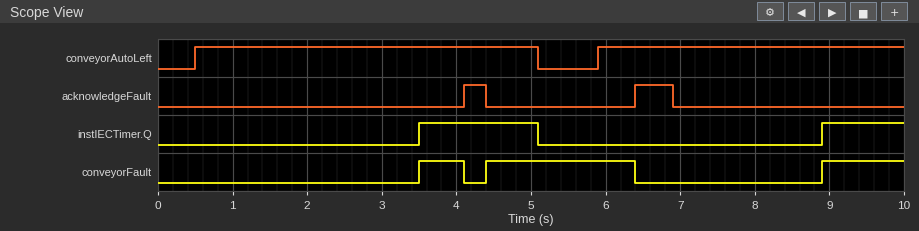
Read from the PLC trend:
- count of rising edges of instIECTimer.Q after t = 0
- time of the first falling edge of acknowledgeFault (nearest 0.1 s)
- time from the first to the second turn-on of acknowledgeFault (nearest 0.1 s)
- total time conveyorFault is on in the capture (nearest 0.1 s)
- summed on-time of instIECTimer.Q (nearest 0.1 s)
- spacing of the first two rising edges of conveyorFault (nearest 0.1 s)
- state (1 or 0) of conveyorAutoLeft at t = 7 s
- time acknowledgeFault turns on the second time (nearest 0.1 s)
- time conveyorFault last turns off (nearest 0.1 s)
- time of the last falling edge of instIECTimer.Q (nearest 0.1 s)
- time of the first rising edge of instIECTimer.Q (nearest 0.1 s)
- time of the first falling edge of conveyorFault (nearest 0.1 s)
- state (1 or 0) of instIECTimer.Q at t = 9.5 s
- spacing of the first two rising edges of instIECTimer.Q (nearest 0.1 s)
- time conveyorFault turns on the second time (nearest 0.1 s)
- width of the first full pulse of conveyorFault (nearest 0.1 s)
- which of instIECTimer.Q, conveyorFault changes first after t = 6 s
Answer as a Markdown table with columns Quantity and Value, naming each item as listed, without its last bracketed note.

| Quantity | Value |
|---|---|
| count of rising edges of instIECTimer.Q after t = 0 | 2 |
| time of the first falling edge of acknowledgeFault | 4.4 s |
| time from the first to the second turn-on of acknowledgeFault | 2.3 s |
| total time conveyorFault is on in the capture | 3.7 s |
| summed on-time of instIECTimer.Q | 2.7 s |
| spacing of the first two rising edges of conveyorFault | 0.9 s |
| state (1 or 0) of conveyorAutoLeft at t = 7 s | 1 |
| time acknowledgeFault turns on the second time | 6.4 s |
| time conveyorFault last turns off | 6.4 s |
| time of the last falling edge of instIECTimer.Q | 5.1 s |
| time of the first rising edge of instIECTimer.Q | 3.5 s |
| time of the first falling edge of conveyorFault | 4.1 s |
| state (1 or 0) of instIECTimer.Q at t = 9.5 s | 1 |
| spacing of the first two rising edges of instIECTimer.Q | 5.4 s |
| time conveyorFault turns on the second time | 4.4 s |
| width of the first full pulse of conveyorFault | 0.6 s |
| which of instIECTimer.Q, conveyorFault changes first after t = 6 s | conveyorFault |
